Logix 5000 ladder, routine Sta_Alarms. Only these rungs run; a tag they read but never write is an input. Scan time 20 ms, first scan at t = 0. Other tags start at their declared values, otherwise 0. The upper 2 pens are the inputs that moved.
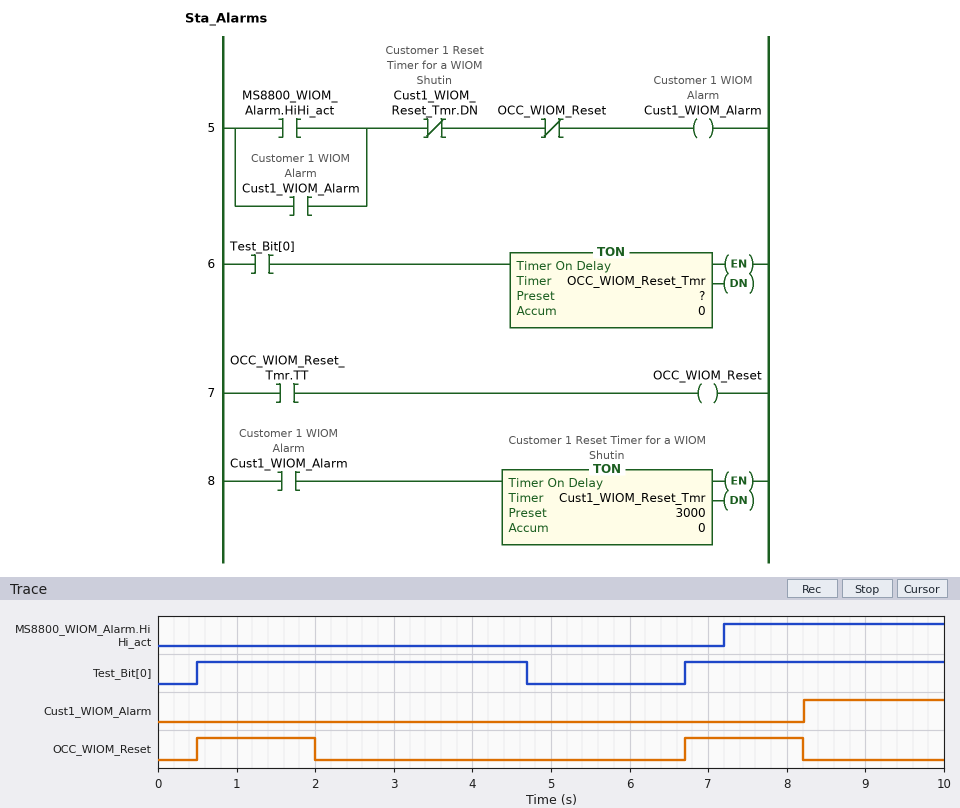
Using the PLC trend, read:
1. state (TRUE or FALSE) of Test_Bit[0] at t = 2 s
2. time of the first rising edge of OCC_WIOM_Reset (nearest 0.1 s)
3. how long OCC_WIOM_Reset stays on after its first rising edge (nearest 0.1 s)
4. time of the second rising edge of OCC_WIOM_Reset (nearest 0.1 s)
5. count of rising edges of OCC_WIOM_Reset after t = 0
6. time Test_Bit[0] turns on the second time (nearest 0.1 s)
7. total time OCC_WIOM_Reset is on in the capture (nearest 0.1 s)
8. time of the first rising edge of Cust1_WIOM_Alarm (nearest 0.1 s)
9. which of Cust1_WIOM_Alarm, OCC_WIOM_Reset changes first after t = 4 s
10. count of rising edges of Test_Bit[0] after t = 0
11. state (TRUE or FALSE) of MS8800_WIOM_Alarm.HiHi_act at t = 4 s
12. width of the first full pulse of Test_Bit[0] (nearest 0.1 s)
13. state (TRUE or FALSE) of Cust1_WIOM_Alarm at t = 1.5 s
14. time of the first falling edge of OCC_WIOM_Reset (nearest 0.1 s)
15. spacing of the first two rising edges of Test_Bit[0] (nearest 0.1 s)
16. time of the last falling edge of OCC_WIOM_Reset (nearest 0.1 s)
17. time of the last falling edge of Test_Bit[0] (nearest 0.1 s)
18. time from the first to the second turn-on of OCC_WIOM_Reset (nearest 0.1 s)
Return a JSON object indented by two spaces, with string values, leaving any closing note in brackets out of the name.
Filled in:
{
  "state (TRUE or FALSE) of Test_Bit[0] at t = 2 s": "TRUE",
  "time of the first rising edge of OCC_WIOM_Reset": "0.5 s",
  "how long OCC_WIOM_Reset stays on after its first rising edge": "1.5 s",
  "time of the second rising edge of OCC_WIOM_Reset": "6.7 s",
  "count of rising edges of OCC_WIOM_Reset after t = 0": "2",
  "time Test_Bit[0] turns on the second time": "6.7 s",
  "total time OCC_WIOM_Reset is on in the capture": "3.0 s",
  "time of the first rising edge of Cust1_WIOM_Alarm": "8.2 s",
  "which of Cust1_WIOM_Alarm, OCC_WIOM_Reset changes first after t = 4 s": "OCC_WIOM_Reset",
  "count of rising edges of Test_Bit[0] after t = 0": "2",
  "state (TRUE or FALSE) of MS8800_WIOM_Alarm.HiHi_act at t = 4 s": "FALSE",
  "width of the first full pulse of Test_Bit[0]": "4.2 s",
  "state (TRUE or FALSE) of Cust1_WIOM_Alarm at t = 1.5 s": "FALSE",
  "time of the first falling edge of OCC_WIOM_Reset": "2.0 s",
  "spacing of the first two rising edges of Test_Bit[0]": "6.2 s",
  "time of the last falling edge of OCC_WIOM_Reset": "8.2 s",
  "time of the last falling edge of Test_Bit[0]": "4.7 s",
  "time from the first to the second turn-on of OCC_WIOM_Reset": "6.2 s"
}
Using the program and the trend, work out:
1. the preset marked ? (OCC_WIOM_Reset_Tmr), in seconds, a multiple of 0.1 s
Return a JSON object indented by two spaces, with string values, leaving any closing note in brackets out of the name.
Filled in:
{
  "the preset marked ? (OCC_WIOM_Reset_Tmr), in seconds, a multiple of 0.1 s": "1.5 s"
}
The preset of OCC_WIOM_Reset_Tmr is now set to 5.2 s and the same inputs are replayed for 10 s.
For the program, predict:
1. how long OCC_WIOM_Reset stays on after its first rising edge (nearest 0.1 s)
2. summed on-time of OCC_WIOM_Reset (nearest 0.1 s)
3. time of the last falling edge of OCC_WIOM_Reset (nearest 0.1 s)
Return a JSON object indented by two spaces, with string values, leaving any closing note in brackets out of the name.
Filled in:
{
  "how long OCC_WIOM_Reset stays on after its first rising edge": "4.2 s",
  "summed on-time of OCC_WIOM_Reset": "7.5 s",
  "time of the last falling edge of OCC_WIOM_Reset": "4.7 s"
}
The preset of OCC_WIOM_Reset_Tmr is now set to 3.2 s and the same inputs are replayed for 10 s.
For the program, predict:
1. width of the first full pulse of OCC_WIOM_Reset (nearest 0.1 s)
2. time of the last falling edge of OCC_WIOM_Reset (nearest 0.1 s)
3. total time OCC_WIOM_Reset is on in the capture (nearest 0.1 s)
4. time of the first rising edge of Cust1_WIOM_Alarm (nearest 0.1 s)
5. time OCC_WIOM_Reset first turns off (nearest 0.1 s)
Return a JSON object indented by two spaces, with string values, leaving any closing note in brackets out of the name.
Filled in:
{
  "width of the first full pulse of OCC_WIOM_Reset": "3.2 s",
  "time of the last falling edge of OCC_WIOM_Reset": "9.9 s",
  "total time OCC_WIOM_Reset is on in the capture": "6.4 s",
  "time of the first rising edge of Cust1_WIOM_Alarm": "9.9 s",
  "time OCC_WIOM_Reset first turns off": "3.7 s"
}
